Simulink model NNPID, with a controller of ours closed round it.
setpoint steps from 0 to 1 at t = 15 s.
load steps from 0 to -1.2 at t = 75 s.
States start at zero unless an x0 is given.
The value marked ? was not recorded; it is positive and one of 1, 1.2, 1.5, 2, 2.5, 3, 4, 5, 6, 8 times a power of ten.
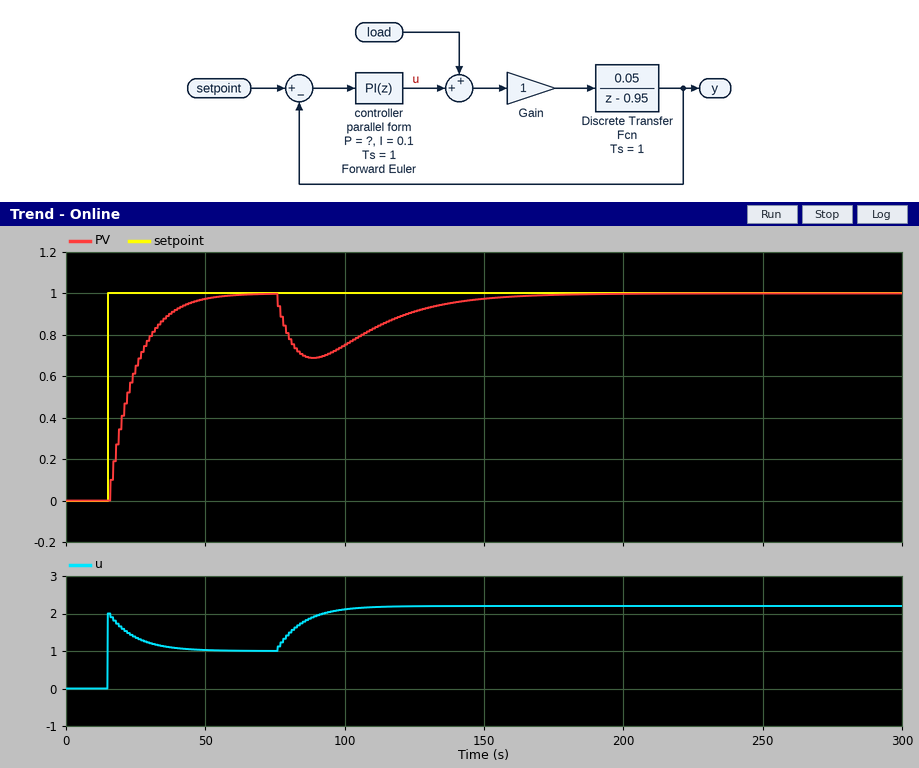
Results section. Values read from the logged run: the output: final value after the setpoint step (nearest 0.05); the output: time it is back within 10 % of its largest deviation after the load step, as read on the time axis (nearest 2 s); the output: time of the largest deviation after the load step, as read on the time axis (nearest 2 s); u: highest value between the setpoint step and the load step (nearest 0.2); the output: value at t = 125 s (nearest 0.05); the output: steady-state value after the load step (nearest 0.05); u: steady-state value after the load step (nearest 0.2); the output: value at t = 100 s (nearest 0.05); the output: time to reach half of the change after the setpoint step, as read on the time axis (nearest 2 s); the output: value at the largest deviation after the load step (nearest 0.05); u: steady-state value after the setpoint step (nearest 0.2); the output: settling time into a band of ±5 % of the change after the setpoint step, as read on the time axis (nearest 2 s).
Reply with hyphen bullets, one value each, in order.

- 1.00
- 146 s
- 88 s
- 2.0
- 0.90
- 1.00
- 2.2
- 0.75
- 22 s
- 0.70
- 1.0
- 44 s
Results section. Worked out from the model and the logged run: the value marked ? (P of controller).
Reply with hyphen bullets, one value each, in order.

- 2
